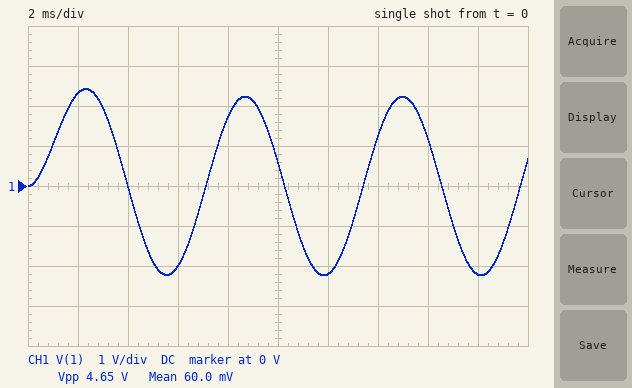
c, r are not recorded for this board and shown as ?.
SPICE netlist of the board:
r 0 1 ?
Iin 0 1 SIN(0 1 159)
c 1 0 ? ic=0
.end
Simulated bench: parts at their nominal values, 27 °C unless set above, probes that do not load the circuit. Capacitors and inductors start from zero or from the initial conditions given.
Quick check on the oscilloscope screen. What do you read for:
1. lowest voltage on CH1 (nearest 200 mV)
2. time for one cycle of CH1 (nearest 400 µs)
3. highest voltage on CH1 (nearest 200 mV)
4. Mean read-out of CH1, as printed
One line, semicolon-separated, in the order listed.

-2.2 V; 6.4 ms; 2.4 V; 60.0 mV
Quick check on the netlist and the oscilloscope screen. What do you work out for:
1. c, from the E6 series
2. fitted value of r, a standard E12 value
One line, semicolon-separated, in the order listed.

330 µF; 3.3 Ω
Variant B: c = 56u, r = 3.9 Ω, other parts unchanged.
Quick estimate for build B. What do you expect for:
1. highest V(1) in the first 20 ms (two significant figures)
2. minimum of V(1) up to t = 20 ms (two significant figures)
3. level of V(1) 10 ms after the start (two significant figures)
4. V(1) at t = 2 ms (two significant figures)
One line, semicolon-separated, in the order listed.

3.8 V; -3.8 V; -1.3 V; 3.7 V
